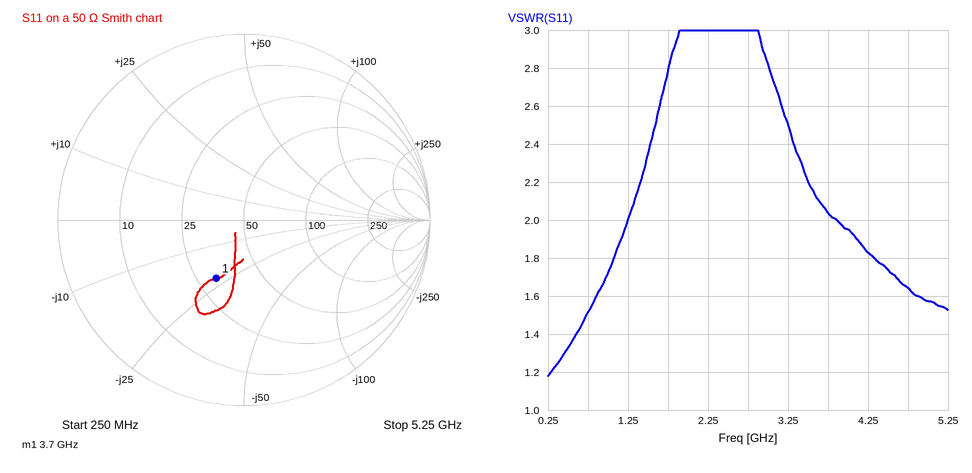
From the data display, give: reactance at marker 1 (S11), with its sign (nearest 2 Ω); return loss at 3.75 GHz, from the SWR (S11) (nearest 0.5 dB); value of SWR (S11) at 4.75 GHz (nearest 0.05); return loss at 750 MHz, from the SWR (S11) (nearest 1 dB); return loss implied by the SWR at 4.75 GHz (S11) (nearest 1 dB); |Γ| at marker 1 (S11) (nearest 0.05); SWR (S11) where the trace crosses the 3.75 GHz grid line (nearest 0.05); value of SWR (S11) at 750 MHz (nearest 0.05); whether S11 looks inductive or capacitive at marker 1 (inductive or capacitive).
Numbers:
-22 Ω
9.5 dB
1.65
14 dB
12 dB
0.35
2.05
1.50
capacitive
